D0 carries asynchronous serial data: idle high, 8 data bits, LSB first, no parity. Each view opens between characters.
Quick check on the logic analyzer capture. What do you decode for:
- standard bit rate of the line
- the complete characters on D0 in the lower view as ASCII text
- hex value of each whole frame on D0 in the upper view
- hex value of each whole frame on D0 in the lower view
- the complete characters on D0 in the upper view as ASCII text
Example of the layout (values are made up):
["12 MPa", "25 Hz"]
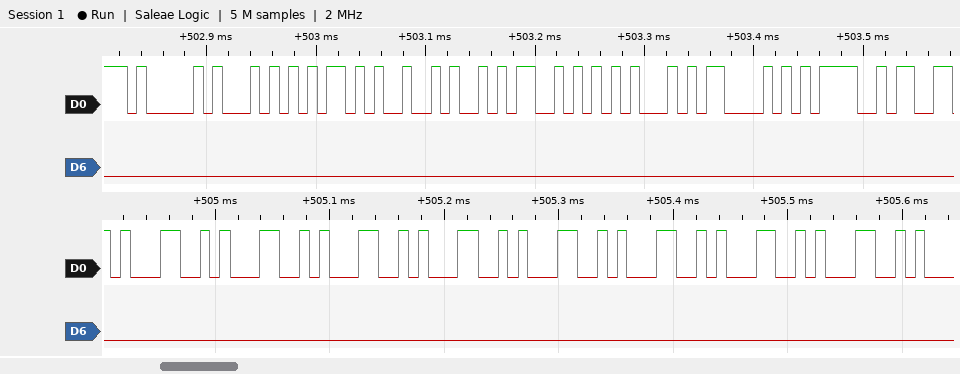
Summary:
["115200 baud", "\"11111111\"", "41, 54, 2B, 4A, 53, 45, 43, 3D", "31, 31, 31, 31, 31, 31, 31, 31", "\"AT+JSEC=\""]
